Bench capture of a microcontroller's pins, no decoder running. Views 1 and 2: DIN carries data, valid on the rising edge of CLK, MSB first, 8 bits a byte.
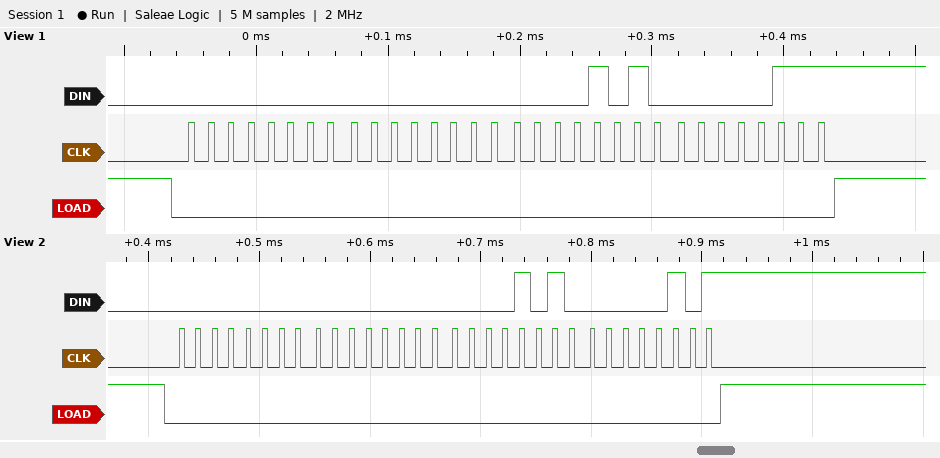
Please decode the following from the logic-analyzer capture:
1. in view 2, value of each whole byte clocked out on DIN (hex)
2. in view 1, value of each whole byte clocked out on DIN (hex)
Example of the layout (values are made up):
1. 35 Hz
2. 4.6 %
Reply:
1. 0x00 0x00 0x0A 0x05
2. 00 00 0A 07
